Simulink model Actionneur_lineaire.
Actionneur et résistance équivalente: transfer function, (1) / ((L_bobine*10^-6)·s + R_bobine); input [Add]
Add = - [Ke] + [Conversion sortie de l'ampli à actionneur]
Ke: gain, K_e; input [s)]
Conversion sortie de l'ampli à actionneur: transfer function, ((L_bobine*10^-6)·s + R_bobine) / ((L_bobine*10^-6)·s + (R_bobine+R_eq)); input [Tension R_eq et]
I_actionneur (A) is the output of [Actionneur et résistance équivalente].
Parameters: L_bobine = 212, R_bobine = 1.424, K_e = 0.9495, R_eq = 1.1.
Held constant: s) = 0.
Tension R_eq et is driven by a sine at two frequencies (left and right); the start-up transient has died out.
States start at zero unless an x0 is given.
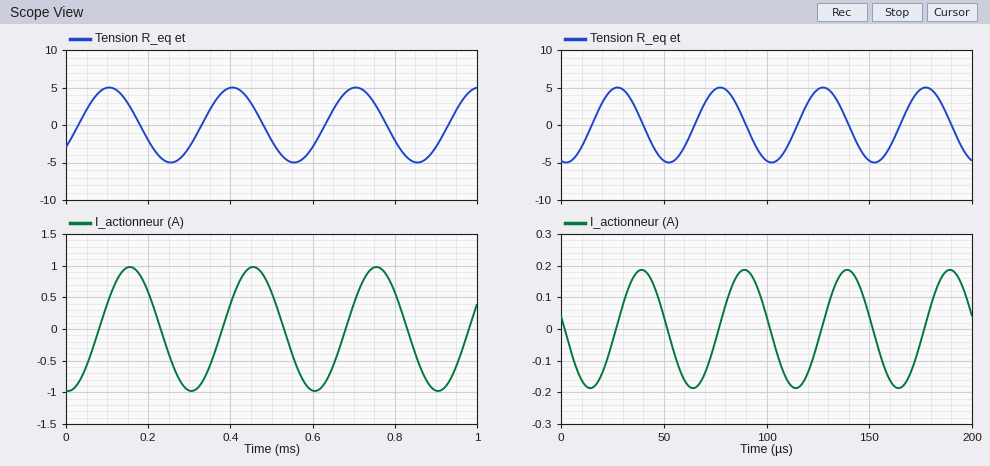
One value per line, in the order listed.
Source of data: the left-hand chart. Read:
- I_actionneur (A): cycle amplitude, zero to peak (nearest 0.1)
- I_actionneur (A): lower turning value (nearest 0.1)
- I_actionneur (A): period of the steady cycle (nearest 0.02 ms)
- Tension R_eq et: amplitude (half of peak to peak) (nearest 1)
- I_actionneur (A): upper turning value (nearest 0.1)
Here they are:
1.0
-1.0
0.30 ms
5
1.0
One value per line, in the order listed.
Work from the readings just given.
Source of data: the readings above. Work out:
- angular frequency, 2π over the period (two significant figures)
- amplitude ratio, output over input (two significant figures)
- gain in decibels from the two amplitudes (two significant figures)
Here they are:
21 rad/ms
0.20
-14 dB
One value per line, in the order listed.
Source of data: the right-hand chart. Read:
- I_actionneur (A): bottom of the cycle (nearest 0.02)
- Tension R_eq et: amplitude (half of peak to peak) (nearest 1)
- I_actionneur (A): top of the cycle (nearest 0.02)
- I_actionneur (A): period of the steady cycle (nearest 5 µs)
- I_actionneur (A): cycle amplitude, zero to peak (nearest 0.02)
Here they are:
-0.18
5
0.18
50 µs
0.18
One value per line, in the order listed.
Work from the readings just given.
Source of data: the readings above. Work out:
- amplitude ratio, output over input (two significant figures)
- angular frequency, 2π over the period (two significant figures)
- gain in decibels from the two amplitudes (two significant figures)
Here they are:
0.036
0.13 rad/µs
-29 dB
